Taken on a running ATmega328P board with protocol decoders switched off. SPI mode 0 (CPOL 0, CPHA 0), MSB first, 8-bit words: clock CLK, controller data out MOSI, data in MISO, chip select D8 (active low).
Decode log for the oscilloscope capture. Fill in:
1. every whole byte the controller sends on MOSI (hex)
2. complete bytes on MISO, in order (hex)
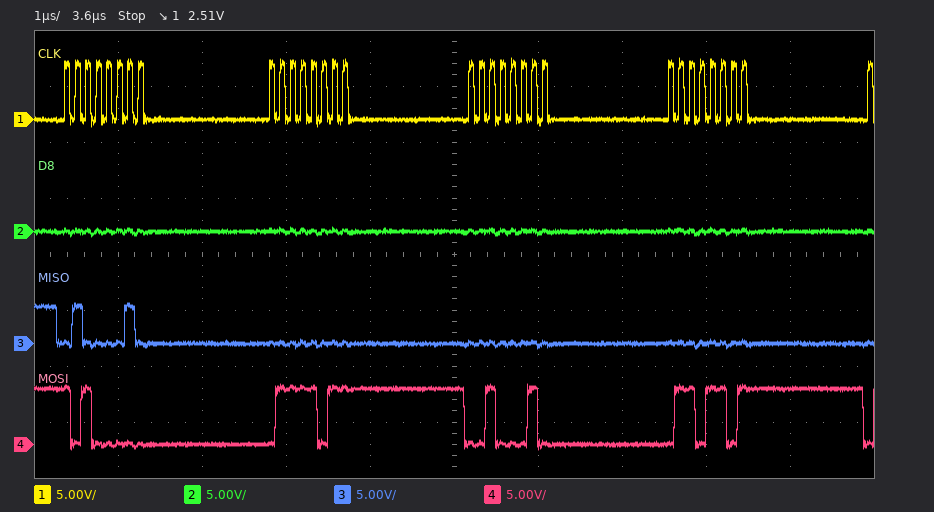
A0 7B 22 6D
42 00 00 00
